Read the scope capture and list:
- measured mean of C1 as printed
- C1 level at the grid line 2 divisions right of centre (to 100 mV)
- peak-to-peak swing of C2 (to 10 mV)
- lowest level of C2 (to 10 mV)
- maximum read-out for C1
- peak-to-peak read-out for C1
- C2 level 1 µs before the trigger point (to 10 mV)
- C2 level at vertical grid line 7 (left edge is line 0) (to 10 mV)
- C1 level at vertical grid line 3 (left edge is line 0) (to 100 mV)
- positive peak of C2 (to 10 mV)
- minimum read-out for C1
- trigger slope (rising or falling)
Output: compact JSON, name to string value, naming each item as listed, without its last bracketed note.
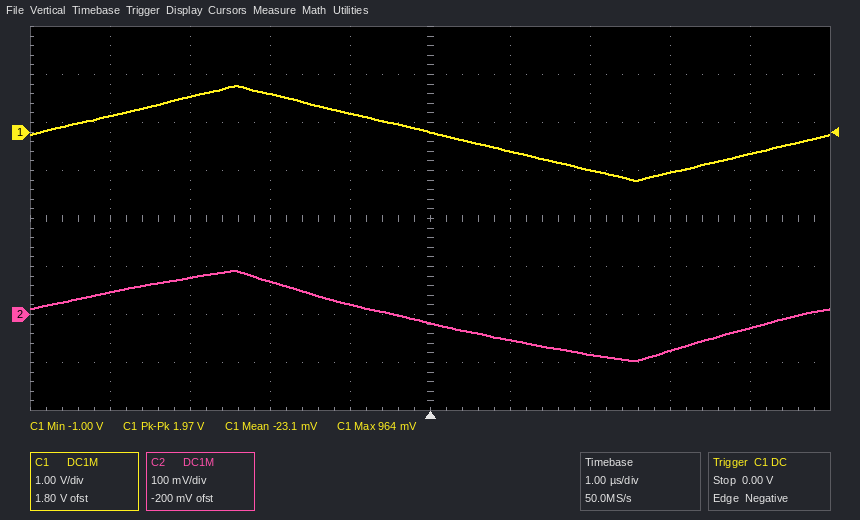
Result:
{"measured mean of C1 as printed": "-23.1 mV", "C1 level at the grid line 2 divisions right of centre": "-800 mV", "peak-to-peak swing of C2": "190 mV", "lowest level of C2": "-100 mV", "maximum read-out for C1": "964 mV", "peak-to-peak read-out for C1": "1.97 V", "C2 level 1 µs before the trigger point": "20 mV", "C2 level at vertical grid line 7 (left edge is line 0)": "-80 mV", "C1 level at vertical grid line 3 (left edge is line 0)": "800 mV", "positive peak of C2": "90 mV", "minimum read-out for C1": "-1.00 V", "trigger slope": "falling"}
